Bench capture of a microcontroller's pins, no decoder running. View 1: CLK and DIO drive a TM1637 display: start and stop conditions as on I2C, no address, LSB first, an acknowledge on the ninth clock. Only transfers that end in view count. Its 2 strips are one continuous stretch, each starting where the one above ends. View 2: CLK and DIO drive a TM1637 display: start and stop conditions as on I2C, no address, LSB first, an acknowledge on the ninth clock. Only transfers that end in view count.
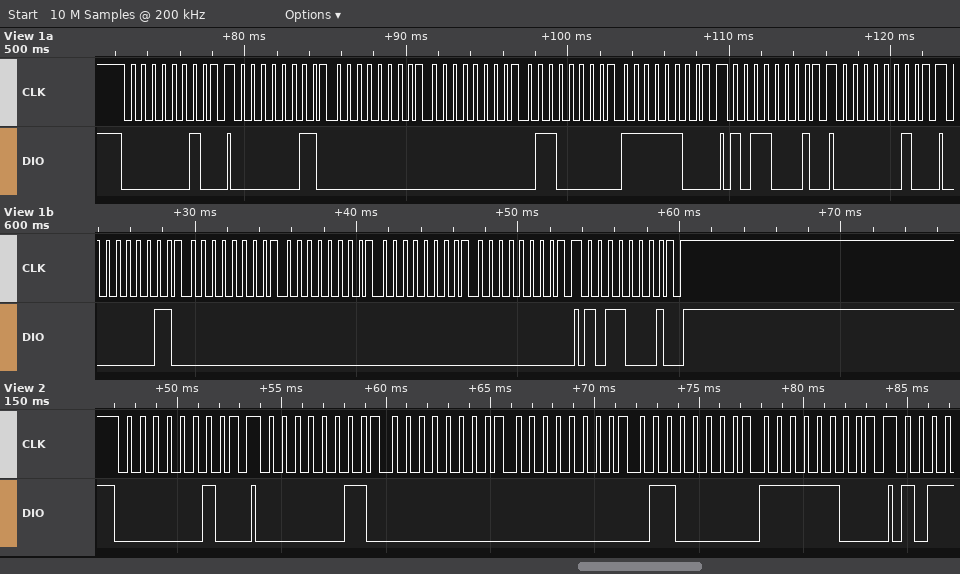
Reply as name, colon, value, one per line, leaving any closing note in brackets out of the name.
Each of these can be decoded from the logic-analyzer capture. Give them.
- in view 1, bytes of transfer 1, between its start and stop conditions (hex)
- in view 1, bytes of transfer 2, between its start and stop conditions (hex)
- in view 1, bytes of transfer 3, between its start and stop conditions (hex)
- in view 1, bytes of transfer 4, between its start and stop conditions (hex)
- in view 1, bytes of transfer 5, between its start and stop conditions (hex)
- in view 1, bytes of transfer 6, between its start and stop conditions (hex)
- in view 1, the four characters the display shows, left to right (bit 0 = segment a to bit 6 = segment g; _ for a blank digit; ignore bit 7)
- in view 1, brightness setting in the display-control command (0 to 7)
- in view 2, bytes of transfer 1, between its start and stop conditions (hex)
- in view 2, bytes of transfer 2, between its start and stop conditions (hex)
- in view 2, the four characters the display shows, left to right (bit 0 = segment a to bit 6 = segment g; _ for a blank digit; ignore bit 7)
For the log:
in view 1, bytes of transfer 1, between its start and stop conditions: 40
in view 1, bytes of transfer 2, between its start and stop conditions: C0 00 00 06 3F
in view 1, bytes of transfer 3, between its start and stop conditions: 8D
in view 1, bytes of transfer 4, between its start and stop conditions: 40
in view 1, bytes of transfer 5, between its start and stop conditions: C0 00 00 00 00
in view 1, bytes of transfer 6, between its start and stop conditions: 8D
in view 1, the four characters the display shows, left to right: ____
in view 1, brightness setting in the display-control command: 5
in view 2, bytes of transfer 1, between its start and stop conditions: 40
in view 2, bytes of transfer 2, between its start and stop conditions: C0 00 00 06 3F
in view 2, the four characters the display shows, left to right: __10
